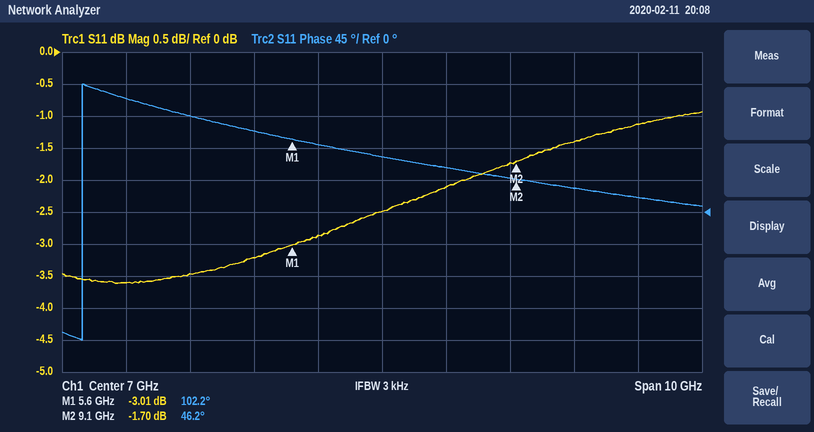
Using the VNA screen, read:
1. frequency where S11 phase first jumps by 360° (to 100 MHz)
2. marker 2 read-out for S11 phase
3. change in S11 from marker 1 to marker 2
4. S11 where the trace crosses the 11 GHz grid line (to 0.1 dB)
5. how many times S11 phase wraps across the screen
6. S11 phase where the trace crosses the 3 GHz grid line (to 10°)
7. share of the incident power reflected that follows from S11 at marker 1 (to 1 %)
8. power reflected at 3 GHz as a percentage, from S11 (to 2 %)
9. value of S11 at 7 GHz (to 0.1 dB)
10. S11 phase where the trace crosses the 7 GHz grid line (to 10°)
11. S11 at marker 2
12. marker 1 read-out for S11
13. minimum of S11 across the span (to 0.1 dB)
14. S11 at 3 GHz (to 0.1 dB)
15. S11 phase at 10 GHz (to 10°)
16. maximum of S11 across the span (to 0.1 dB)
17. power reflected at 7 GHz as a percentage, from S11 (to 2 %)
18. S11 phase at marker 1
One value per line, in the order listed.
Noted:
2.3 GHz
46.2°
1.31 dB
-1.1 dB
1
160°
50 %
44 %
-2.5 dB
80°
-1.70 dB
-3.01 dB
-3.6 dB
-3.6 dB
30°
-0.9 dB
56 %
102.2°
